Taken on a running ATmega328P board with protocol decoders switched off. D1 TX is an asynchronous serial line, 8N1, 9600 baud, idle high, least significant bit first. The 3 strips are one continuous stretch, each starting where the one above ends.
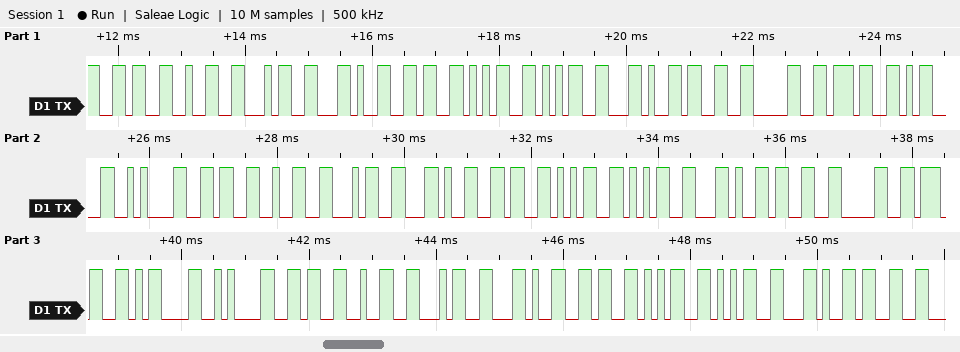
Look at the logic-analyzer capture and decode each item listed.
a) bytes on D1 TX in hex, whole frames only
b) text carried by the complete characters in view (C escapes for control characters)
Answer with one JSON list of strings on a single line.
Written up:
["36 32 34 2C 36 35 35 2C 33 30 37 0D 0A 36 32 34 2C 36 35 35 2C 33 30 37 0D 0A 36 32 34 2C 36 35 35 2C 33", "\"624,655,307\\r\\n624,655,307\\r\\n624,655,3\""]
